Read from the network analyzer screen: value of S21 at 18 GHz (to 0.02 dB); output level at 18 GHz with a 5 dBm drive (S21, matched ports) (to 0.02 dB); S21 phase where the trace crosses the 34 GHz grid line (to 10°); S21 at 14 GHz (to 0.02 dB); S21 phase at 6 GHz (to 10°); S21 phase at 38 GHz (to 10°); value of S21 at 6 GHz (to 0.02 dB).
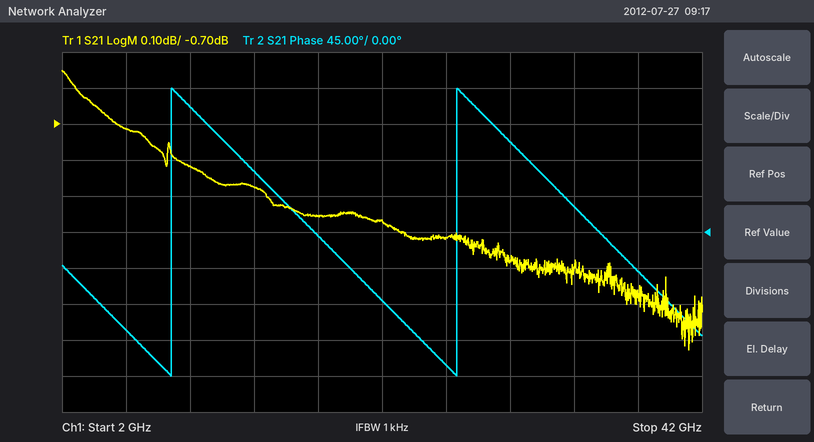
-0.96 dB
4.04 dBm
30°
-0.88 dB
-120°
-50°
-0.72 dB
